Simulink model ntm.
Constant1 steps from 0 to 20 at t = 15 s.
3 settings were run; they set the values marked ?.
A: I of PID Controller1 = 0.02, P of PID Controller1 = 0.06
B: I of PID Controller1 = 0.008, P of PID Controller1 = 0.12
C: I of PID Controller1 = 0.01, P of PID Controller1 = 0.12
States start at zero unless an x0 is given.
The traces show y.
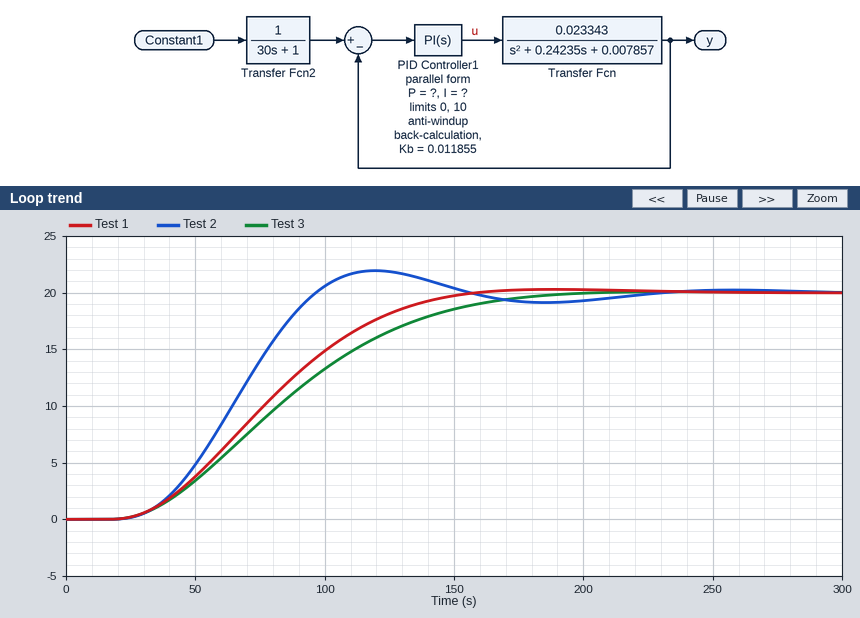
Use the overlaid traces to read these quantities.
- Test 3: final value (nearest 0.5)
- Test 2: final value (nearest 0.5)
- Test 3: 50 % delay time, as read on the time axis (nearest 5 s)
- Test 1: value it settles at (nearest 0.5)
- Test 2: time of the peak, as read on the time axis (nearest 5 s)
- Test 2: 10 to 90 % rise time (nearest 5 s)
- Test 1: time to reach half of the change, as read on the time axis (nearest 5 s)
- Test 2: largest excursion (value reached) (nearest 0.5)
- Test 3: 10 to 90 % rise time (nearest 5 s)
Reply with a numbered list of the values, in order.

1. 20.0
2. 20.0
3. 80 s
4. 20.0
5. 120 s
6. 50 s
7. 75 s
8. 22.0
9. 100 s
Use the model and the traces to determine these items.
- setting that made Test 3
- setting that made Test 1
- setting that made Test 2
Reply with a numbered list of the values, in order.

1. B
2. C
3. A
